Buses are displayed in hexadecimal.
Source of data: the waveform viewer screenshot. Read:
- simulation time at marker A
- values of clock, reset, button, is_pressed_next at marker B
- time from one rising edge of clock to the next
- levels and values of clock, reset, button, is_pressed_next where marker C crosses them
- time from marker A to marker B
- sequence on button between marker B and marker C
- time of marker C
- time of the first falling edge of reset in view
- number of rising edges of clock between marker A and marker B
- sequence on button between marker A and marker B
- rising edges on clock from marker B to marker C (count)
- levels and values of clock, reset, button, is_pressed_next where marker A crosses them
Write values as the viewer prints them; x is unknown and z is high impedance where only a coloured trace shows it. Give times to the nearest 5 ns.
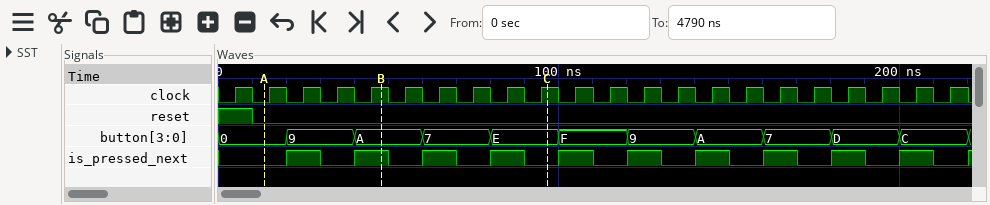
15 ns
clock=1, reset=0, button=A, is_pressed_next=1
10 ns
clock=1, reset=0, button=E, is_pressed_next=0
35 ns
A, 7, E
95 ns
10 ns
4
0, 9, A
5
clock=0, reset=0, button=0, is_pressed_next=0
